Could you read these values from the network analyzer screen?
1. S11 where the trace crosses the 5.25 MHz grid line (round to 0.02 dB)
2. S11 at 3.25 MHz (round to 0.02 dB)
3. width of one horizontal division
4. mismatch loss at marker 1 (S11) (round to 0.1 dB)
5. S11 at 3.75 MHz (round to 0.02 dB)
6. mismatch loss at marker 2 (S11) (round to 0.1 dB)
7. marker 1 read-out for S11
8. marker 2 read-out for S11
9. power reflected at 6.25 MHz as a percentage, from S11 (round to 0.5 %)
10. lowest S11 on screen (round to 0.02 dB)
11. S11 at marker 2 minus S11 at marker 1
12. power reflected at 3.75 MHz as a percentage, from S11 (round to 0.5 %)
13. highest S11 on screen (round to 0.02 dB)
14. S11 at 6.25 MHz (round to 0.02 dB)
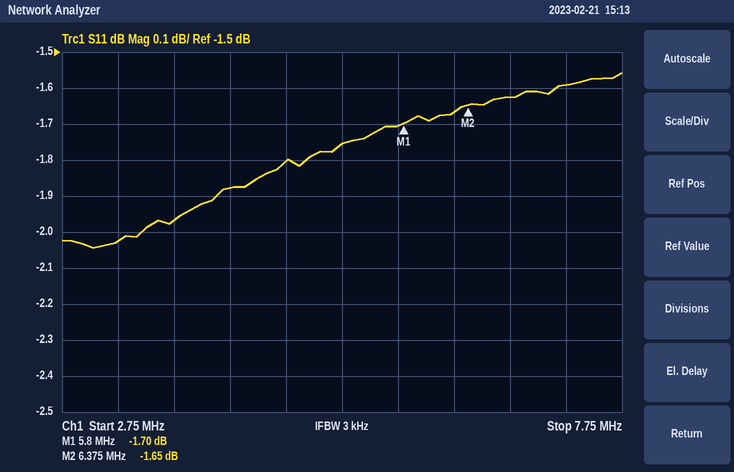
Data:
-1.76 dB
-2.02 dB
500 kHz
4.9 dB
-1.96 dB
5.0 dB
-1.70 dB
-1.65 dB
68.0 %
-2.04 dB
0.05 dB
63.5 %
-1.56 dB
-1.66 dB
